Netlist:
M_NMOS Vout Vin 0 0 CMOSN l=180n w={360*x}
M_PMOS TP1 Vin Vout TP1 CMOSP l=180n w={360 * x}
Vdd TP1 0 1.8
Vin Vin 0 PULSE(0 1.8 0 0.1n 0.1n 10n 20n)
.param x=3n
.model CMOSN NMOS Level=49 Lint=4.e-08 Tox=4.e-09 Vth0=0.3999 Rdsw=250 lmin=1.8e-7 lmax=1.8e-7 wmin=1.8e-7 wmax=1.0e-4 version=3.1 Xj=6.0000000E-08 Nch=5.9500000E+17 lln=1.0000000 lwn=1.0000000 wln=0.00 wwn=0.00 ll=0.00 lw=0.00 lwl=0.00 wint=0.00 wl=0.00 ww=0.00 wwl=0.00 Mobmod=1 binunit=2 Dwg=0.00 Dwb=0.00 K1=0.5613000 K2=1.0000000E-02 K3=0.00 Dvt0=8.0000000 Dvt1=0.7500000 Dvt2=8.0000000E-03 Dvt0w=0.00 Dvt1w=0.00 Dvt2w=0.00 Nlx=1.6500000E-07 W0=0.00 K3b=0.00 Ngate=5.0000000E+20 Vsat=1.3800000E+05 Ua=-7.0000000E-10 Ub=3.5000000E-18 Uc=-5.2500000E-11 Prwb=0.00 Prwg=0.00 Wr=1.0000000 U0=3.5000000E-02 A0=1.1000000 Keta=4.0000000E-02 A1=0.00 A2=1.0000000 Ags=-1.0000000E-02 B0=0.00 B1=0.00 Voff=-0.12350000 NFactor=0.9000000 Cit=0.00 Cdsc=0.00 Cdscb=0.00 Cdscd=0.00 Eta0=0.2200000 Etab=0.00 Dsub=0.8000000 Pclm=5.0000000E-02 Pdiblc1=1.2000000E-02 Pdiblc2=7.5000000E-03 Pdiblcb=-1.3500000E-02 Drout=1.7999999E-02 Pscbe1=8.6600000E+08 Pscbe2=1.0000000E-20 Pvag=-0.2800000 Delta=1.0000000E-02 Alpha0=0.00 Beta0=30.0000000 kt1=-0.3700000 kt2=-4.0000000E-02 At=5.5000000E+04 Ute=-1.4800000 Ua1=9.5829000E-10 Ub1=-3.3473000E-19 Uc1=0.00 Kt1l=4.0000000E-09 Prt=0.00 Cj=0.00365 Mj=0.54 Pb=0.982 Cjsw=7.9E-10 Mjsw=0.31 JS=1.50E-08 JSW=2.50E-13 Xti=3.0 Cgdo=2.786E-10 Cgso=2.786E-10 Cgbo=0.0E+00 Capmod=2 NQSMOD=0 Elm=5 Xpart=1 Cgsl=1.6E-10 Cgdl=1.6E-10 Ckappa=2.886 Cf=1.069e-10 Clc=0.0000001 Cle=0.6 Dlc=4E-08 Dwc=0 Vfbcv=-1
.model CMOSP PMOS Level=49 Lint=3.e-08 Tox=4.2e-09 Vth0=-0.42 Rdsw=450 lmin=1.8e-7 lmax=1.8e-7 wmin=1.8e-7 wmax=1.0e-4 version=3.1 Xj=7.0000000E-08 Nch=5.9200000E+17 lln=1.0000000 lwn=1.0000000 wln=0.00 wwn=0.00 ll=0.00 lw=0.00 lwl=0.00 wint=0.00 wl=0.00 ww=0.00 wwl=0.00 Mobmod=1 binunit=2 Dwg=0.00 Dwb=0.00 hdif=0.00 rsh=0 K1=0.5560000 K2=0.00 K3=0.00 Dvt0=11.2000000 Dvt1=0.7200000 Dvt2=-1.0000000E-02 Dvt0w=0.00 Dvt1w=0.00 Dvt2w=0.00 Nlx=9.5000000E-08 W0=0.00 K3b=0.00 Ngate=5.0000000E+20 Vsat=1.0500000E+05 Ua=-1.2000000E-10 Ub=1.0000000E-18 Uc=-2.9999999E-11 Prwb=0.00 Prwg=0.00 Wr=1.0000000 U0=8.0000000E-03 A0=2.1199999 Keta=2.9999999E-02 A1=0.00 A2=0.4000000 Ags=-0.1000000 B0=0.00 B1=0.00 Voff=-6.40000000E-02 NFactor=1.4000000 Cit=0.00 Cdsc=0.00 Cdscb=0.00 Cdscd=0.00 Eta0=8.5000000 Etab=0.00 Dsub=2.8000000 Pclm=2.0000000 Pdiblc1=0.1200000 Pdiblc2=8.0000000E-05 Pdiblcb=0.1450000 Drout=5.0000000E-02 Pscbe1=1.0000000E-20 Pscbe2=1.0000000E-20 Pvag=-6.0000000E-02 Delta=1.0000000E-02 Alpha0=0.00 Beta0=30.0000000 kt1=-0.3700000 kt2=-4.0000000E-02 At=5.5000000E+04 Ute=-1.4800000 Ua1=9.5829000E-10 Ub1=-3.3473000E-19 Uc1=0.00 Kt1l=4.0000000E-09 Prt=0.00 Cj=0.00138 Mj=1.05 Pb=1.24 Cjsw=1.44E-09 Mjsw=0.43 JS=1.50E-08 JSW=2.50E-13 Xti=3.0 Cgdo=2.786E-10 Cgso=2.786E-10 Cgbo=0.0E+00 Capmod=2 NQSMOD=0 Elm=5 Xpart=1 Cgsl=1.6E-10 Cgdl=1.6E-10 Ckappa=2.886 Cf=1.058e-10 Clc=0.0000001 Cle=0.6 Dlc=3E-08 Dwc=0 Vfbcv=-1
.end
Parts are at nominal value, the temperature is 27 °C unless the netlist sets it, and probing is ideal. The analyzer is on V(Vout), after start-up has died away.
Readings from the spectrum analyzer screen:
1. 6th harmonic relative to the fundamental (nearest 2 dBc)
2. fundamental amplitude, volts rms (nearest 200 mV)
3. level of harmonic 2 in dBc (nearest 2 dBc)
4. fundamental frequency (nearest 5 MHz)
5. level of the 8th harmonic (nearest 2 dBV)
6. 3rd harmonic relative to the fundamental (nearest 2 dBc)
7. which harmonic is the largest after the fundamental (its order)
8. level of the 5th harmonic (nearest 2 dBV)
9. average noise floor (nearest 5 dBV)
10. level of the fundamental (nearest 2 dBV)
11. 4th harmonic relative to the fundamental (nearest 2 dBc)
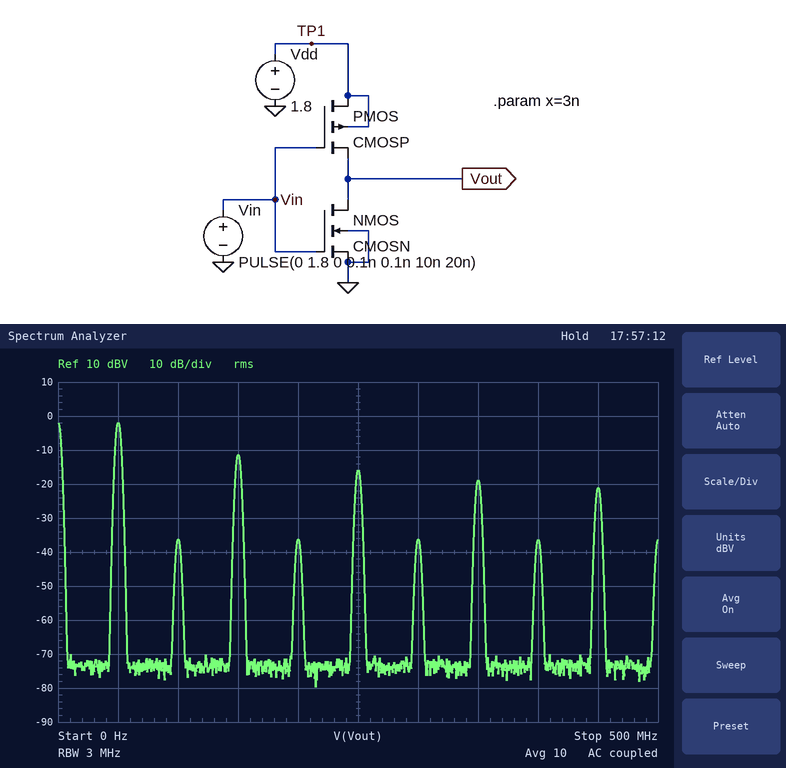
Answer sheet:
-34 dBc
800 mV
-34 dBc
50 MHz
-36 dBV
-10 dBc
3
-16 dBV
-75 dBV
-2 dBV
-34 dBc
